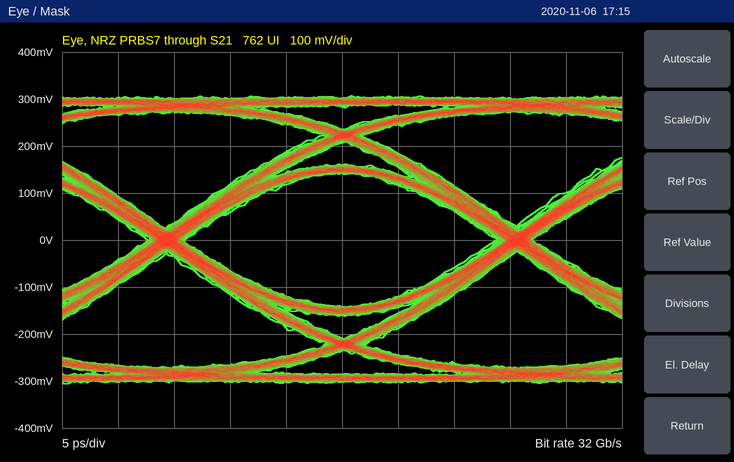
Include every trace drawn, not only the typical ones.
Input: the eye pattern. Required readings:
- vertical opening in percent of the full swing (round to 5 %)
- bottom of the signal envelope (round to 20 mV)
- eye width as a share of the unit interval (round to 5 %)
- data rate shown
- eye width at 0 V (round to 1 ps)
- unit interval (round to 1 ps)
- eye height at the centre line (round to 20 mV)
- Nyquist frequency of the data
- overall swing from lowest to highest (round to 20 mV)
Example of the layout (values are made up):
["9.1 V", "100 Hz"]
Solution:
["45 %", "-300 mV", "90 %", "32 Gb/s", "28 ps", "31 ps", "280 mV", "16 GHz", "620 mV"]
